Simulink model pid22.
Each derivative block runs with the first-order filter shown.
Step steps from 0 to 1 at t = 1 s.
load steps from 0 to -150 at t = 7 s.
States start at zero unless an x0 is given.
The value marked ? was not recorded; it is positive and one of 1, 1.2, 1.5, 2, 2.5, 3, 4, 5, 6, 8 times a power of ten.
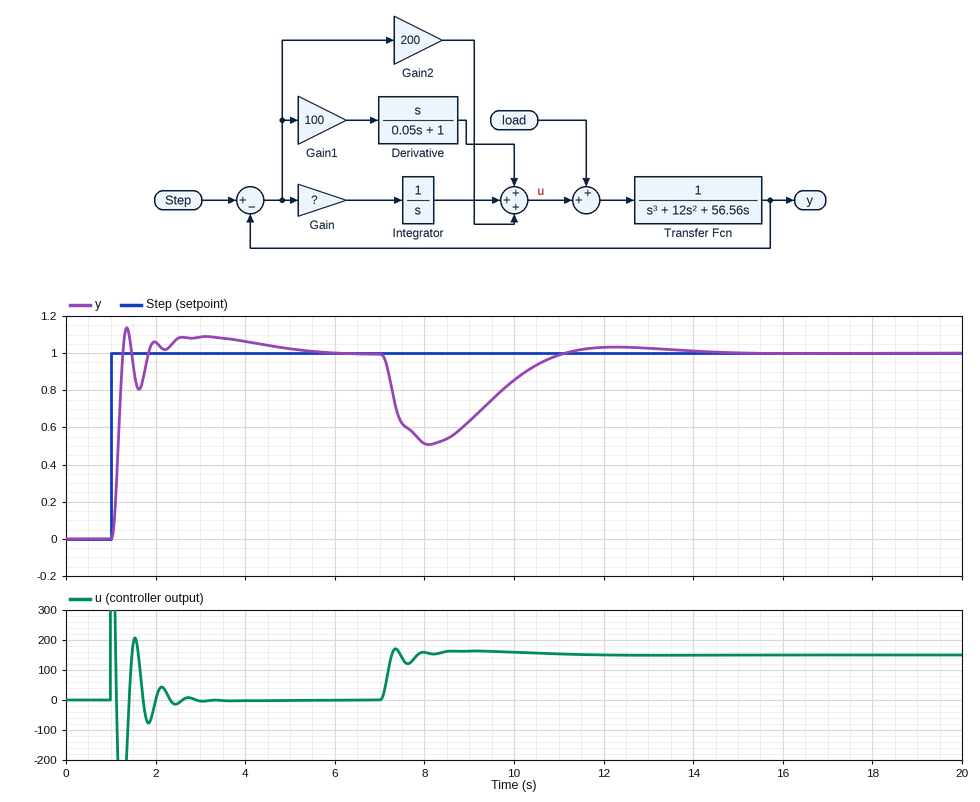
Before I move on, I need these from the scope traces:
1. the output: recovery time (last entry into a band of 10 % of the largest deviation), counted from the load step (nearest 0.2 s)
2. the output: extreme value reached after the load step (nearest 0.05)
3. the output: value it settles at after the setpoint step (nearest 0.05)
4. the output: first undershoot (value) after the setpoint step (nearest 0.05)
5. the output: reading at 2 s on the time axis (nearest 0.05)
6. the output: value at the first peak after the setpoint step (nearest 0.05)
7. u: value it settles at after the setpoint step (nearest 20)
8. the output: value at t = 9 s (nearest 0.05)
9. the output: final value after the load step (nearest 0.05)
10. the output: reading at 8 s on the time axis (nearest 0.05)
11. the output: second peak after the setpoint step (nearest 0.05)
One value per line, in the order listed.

3.6 s
0.50
1.00
0.80
1.05
1.15
0
0.65
1.00
0.50
1.10
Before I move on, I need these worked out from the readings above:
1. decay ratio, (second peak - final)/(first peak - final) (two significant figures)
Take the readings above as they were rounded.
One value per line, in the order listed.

0.67
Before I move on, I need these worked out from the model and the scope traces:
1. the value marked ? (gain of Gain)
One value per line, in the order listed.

150
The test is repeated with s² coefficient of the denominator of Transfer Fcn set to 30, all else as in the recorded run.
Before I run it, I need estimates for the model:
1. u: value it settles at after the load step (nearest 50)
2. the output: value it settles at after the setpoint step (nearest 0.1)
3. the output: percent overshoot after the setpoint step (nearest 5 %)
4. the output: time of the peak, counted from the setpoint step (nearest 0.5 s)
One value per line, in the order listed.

150
1.0
15 %
1.5 s
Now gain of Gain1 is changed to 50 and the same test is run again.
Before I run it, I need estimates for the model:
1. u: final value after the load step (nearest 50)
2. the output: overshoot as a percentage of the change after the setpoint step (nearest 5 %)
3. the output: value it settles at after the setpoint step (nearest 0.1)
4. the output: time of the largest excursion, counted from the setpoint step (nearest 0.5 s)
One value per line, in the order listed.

150
10 %
1.0
1.5 s
